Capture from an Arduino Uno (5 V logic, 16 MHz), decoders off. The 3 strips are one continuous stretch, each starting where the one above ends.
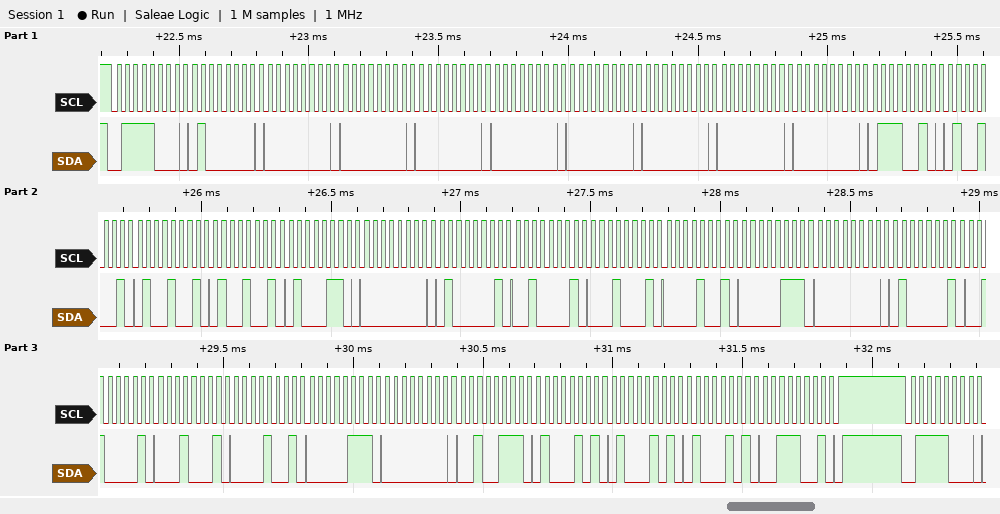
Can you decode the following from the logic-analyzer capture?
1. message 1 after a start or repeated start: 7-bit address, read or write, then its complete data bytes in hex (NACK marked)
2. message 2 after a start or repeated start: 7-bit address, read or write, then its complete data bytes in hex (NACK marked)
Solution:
0x3C write: 40 00 00 00 00 00 00 00 00 72 49 49 49 46 00 41 21 11 09 07 00 41 21 11 09 07 00 27 45 45 45 39
0x3C write
